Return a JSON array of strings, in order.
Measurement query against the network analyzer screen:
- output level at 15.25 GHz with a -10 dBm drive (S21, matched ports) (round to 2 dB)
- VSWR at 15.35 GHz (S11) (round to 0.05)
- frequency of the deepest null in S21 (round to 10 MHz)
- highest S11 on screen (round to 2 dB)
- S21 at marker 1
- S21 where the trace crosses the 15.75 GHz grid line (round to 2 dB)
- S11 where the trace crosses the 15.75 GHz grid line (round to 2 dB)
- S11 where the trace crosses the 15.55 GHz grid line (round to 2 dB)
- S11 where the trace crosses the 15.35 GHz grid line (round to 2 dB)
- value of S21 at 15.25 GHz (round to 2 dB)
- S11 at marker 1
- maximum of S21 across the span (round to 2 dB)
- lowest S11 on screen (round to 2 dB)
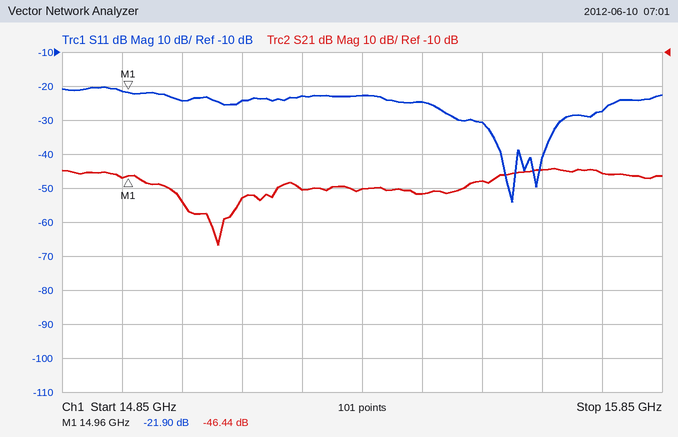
["-60 dBm", "1.15", "15.11 GHz", "-20 dB", "-46.44 dB", "-46 dB", "-28 dB", "-30 dB", "-22 dB", "-50 dB", "-21.90 dB", "-44 dB", "-54 dB"]
